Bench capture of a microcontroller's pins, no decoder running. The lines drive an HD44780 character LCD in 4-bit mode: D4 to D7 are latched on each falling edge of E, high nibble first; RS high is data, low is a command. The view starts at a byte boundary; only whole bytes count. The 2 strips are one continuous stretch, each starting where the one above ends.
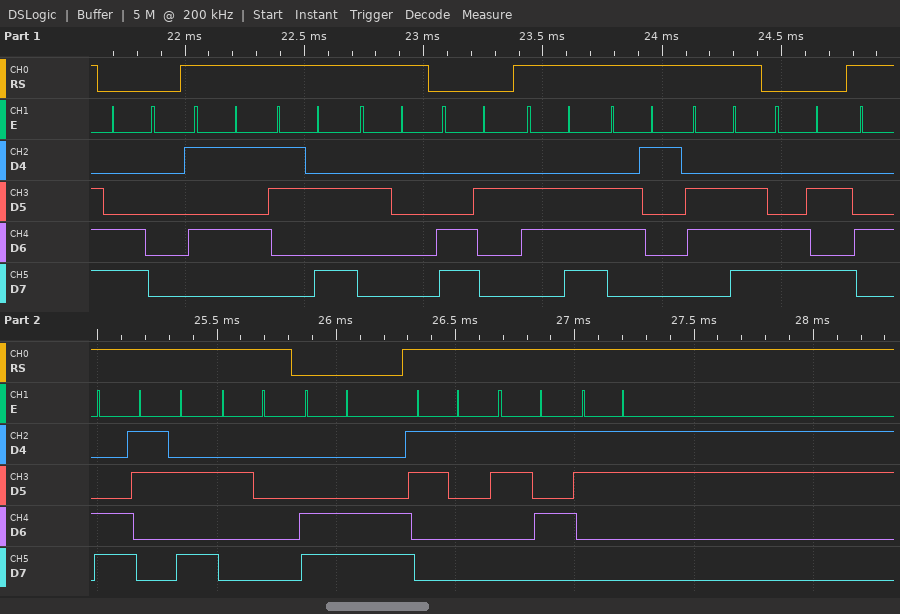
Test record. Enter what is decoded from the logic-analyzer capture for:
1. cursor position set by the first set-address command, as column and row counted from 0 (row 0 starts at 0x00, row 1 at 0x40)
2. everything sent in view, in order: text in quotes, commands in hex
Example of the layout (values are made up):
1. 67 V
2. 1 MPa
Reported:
1. column 0, row 1
2. 0xC0 "U: " 0xC2 "nan" 0xCA "L: " 0xCC "153"
